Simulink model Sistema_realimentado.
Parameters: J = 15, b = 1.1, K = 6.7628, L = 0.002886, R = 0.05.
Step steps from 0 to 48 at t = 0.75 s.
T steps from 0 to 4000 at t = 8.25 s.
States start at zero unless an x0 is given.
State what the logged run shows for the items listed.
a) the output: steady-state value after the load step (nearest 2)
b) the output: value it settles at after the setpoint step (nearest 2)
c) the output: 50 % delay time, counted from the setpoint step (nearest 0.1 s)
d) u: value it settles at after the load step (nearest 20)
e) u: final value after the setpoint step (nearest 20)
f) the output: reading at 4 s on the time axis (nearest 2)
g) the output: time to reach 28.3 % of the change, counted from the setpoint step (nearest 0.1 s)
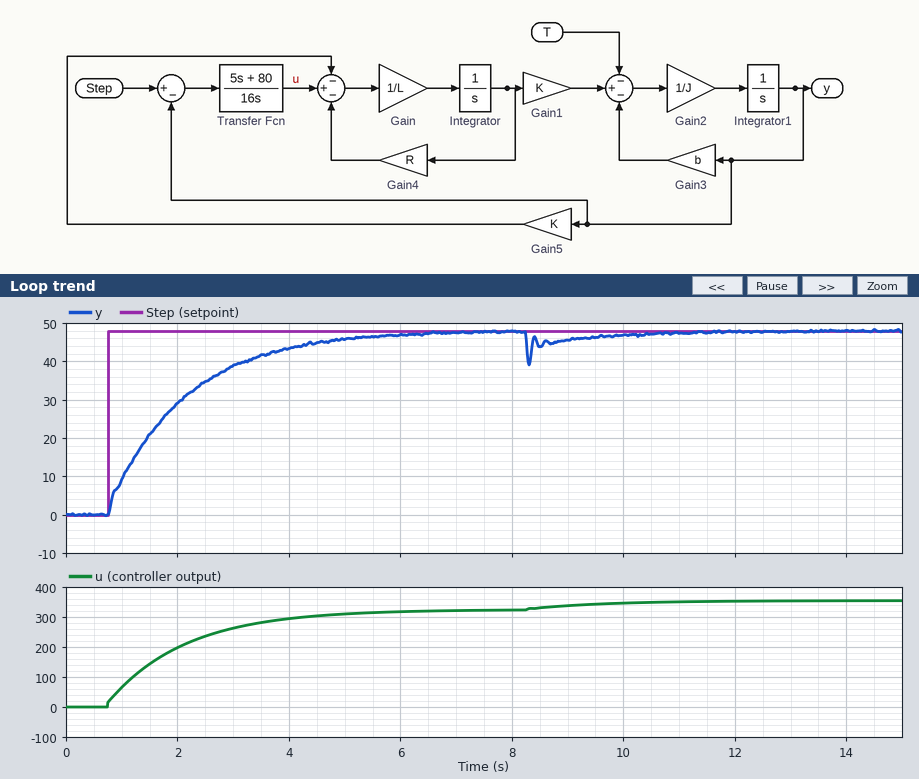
48
48
0.9 s
360
320
44
0.4 s
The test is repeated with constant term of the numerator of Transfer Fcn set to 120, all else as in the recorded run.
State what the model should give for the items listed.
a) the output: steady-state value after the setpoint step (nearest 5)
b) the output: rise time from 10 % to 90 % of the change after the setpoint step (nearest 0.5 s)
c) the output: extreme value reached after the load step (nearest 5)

50
2.0 s
40
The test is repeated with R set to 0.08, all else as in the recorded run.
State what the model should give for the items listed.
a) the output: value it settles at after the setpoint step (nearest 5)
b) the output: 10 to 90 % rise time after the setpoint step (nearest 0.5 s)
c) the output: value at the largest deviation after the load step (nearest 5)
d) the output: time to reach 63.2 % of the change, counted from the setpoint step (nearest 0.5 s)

50
3.0 s
40
1.5 s
